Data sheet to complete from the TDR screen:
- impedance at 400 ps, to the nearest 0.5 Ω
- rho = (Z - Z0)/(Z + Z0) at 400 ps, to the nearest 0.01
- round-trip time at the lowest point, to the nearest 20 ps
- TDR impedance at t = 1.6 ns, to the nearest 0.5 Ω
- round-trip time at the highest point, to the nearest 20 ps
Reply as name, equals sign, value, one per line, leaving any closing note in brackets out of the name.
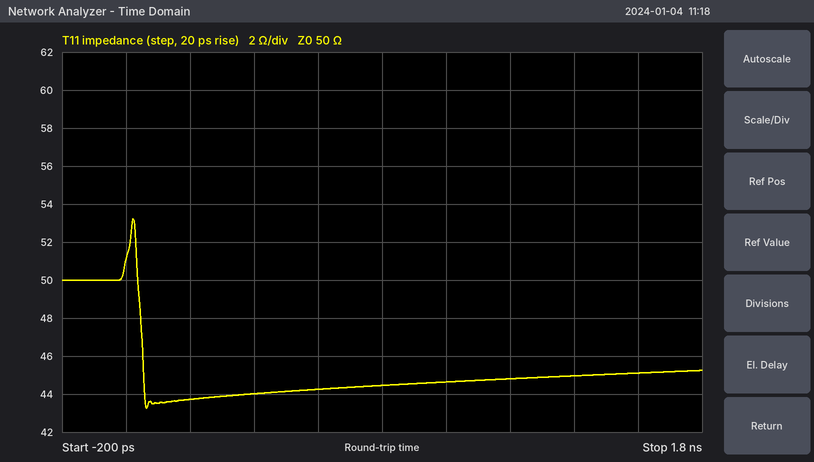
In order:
impedance at 400 ps, to the nearest 0.5 Ω = 44.0 Ω
rho = (Z - Z0)/(Z + Z0) at 400 ps, to the nearest 0.01 = -0.06
round-trip time at the lowest point, to the nearest 20 ps = 60 ps
TDR impedance at t = 1.6 ns, to the nearest 0.5 Ω = 45.0 Ω
round-trip time at the highest point, to the nearest 20 ps = 20 ps
